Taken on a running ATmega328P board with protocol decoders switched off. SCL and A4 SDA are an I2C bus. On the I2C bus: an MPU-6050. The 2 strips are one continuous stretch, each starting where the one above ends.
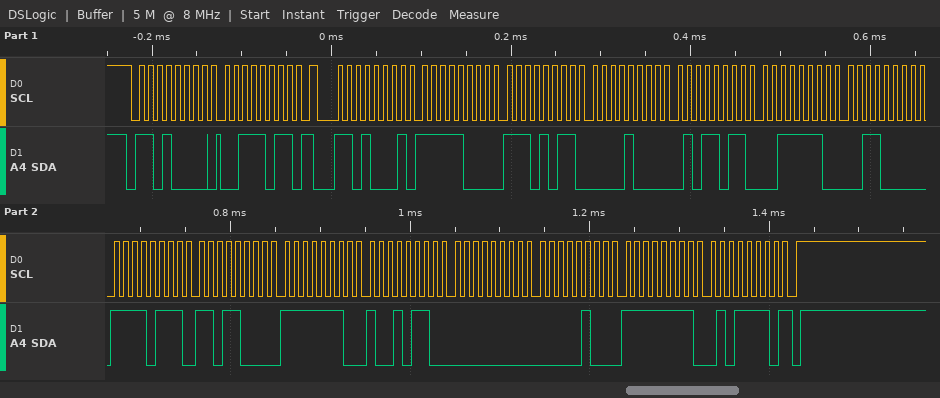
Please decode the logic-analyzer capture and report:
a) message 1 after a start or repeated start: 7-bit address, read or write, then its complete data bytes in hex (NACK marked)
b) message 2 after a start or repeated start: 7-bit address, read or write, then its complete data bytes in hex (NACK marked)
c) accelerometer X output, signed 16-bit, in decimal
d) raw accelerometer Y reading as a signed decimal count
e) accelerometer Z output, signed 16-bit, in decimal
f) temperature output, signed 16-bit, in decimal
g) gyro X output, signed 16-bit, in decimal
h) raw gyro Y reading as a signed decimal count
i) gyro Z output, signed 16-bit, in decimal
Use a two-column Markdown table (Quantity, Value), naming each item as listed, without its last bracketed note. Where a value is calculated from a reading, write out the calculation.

| Quantity | Value |
|---|---|
| message 1 after a start or repeated start: 7-bit address, read or write, then its complete data bytes in hex | 0x68 write: 3B |
| message 2 after a start or repeated start: 7-bit address, read or write, then its complete data bytes in hex | 0x68 read: F8 EB 08 5B 3E 30 F7 D8 FE 96 00 04 FF 5E NACK |
| accelerometer X output, signed 16-bit, in decimal | 0xF8EB = -1813 |
| raw accelerometer Y reading as a signed decimal count | 0x085B = 2139 |
| accelerometer Z output, signed 16-bit, in decimal | 0x3E30 = 15920 |
| temperature output, signed 16-bit, in decimal | 0xF7D8 = -2088 |
| gyro X output, signed 16-bit, in decimal | 0xFE96 = -362 |
| raw gyro Y reading as a signed decimal count | 0x0004 = 4 |
| gyro Z output, signed 16-bit, in decimal | 0xFF5E = -162 |
